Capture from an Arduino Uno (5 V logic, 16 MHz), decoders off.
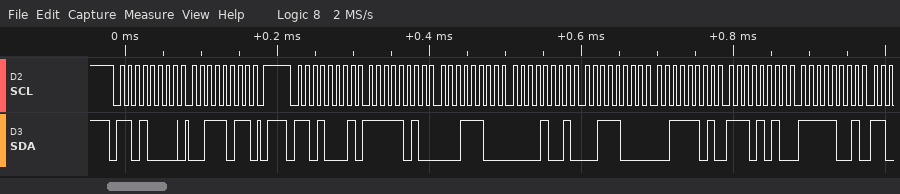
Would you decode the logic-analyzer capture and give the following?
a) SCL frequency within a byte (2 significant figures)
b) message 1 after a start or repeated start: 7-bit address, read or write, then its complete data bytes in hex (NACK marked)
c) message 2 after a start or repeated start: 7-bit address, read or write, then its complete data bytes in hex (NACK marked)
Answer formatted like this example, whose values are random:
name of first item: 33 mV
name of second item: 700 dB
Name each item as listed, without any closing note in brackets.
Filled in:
SCL frequency within a byte: 100 kHz
message 1 after a start or repeated start: 7-bit address, read or write, then its complete data bytes in hex: 0x68 write: 3B
message 2 after a start or repeated start: 7-bit address, read or write, then its complete data bytes in hex: 0x68 read: FA 1C 09 38 3D EA F9
